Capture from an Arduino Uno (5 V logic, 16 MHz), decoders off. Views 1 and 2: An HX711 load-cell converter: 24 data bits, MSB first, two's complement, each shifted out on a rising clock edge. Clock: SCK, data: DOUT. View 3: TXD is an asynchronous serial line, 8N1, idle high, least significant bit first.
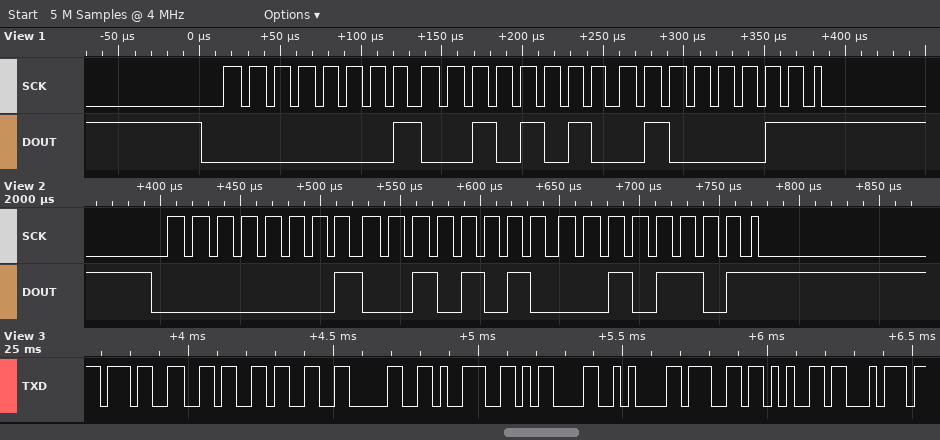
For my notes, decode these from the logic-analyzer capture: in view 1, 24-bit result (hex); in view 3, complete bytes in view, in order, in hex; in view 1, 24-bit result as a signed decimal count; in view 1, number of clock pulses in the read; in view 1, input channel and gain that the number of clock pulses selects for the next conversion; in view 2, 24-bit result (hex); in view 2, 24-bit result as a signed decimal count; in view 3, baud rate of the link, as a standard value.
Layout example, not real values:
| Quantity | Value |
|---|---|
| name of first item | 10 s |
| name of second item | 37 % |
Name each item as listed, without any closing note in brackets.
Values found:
| Quantity | Value |
|---|---|
| in view 1, 24-bit result | 0x012A43 |
| in view 3, complete bytes in view, in order, in hex | 37 36 33 30 39 0D 0A 67 65 74 |
| in view 1, 24-bit result as a signed decimal count | 76355 |
| in view 1, number of clock pulses in the read | 25 |
| in view 1, input channel and gain that the number of clock pulses selects for the next conversion | channel A, gain 128 |
| in view 2, 24-bit result | 0x012A2D |
| in view 2, 24-bit result as a signed decimal count | 76333 |
| in view 3, baud rate of the link, as a standard value | 38400 baud |
